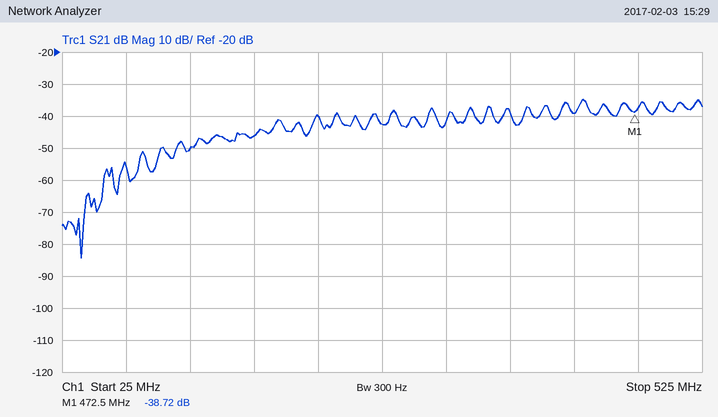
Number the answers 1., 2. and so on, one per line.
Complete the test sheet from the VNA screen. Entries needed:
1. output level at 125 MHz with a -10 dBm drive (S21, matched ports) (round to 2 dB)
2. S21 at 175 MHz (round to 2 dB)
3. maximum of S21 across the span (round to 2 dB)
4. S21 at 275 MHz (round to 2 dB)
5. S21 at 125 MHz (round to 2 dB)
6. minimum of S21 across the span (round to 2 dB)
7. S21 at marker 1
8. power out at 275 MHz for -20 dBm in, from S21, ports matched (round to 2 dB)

1. -60 dBm
2. -46 dB
3. -34 dB
4. -42 dB
5. -50 dB
6. -84 dB
7. -38.72 dB
8. -62 dBm
